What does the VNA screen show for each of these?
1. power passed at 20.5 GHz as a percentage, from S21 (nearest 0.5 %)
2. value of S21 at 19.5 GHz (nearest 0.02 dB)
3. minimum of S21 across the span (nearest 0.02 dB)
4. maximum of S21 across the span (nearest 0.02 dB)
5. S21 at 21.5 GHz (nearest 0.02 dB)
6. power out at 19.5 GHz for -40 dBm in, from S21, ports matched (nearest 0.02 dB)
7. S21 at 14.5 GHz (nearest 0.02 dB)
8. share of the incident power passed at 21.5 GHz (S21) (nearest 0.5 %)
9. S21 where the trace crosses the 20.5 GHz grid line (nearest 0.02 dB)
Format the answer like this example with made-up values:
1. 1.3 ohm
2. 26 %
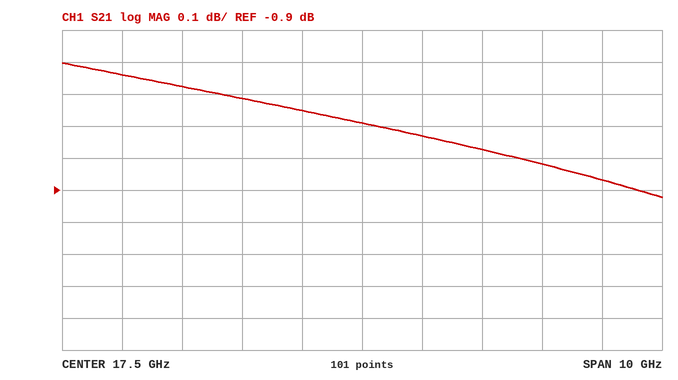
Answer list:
1. 83.0 %
2. -0.78 dB
3. -0.92 dB
4. -0.50 dB
5. -0.86 dB
6. -40.78 dBm
7. -0.58 dB
8. 82.0 %
9. -0.82 dB
